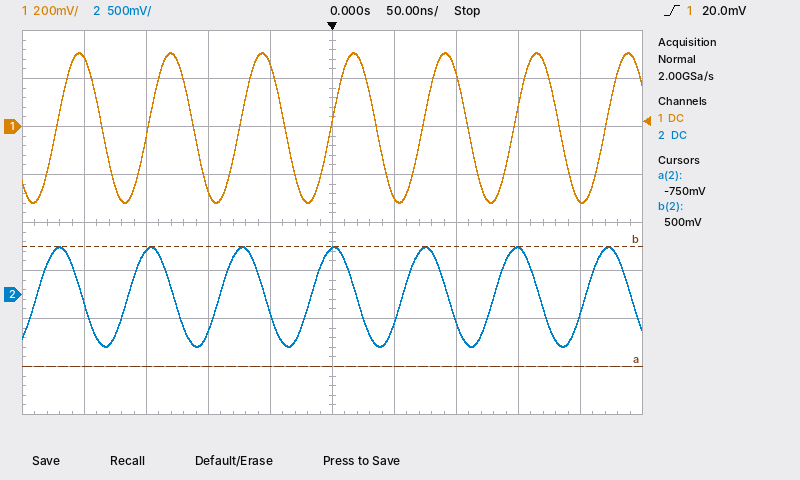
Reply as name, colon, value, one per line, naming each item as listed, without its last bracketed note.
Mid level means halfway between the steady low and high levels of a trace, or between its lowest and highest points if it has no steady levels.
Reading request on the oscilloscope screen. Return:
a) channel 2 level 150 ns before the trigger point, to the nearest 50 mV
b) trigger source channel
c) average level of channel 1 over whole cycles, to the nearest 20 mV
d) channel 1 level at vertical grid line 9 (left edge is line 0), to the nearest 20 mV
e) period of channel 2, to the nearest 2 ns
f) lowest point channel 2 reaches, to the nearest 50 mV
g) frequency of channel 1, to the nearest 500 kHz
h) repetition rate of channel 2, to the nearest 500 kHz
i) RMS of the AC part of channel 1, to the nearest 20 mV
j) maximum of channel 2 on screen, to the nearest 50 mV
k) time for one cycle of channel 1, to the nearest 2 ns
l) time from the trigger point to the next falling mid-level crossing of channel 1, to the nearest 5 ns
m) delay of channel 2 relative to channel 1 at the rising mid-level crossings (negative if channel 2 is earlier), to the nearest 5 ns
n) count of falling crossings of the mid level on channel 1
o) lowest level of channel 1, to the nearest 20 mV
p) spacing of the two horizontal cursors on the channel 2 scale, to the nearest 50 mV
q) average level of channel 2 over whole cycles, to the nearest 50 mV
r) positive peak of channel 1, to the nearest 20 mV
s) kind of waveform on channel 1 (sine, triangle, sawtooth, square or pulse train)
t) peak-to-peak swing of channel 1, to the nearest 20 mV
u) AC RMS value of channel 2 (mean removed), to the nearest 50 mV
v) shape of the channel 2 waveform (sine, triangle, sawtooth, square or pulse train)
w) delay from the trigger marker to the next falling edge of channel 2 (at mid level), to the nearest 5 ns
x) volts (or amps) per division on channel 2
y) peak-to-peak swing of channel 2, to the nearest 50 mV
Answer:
channel 2 level 150 ns before the trigger point, to the nearest 50 mV: 450 mV
trigger source channel: channel 1
average level of channel 1 over whole cycles, to the nearest 20 mV: 0 mV
channel 1 level at vertical grid line 9 (left edge is line 0), to the nearest 20 mV: -300 mV
period of channel 2, to the nearest 2 ns: 74 ns
lowest point channel 2 reaches, to the nearest 50 mV: -550 mV
frequency of channel 1, to the nearest 500 kHz: 13.5 MHz
repetition rate of channel 2, to the nearest 500 kHz: 13.5 MHz
RMS of the AC part of channel 1, to the nearest 20 mV: 220 mV
maximum of channel 2 on screen, to the nearest 50 mV: 500 mV
time for one cycle of channel 1, to the nearest 2 ns: 74 ns
time from the trigger point to the next falling mid-level crossing of channel 1, to the nearest 5 ns: 35 ns
delay of channel 2 relative to channel 1 at the rising mid-level crossings (negative if channel 2 is earlier), to the nearest 5 ns: -15 ns
count of falling crossings of the mid level on channel 1: 6
lowest level of channel 1, to the nearest 20 mV: -320 mV
spacing of the two horizontal cursors on the channel 2 scale, to the nearest 50 mV: 1.25 V
average level of channel 2 over whole cycles, to the nearest 50 mV: 0 mV
positive peak of channel 1, to the nearest 20 mV: 300 mV
kind of waveform on channel 1: sine
peak-to-peak swing of channel 1, to the nearest 20 mV: 620 mV
AC RMS value of channel 2 (mean removed), to the nearest 50 mV: 350 mV
shape of the channel 2 waveform: sine
delay from the trigger marker to the next falling edge of channel 2 (at mid level), to the nearest 5 ns: 20 ns
volts (or amps) per division on channel 2: 500 mV
peak-to-peak swing of channel 2, to the nearest 50 mV: 1.05 V
